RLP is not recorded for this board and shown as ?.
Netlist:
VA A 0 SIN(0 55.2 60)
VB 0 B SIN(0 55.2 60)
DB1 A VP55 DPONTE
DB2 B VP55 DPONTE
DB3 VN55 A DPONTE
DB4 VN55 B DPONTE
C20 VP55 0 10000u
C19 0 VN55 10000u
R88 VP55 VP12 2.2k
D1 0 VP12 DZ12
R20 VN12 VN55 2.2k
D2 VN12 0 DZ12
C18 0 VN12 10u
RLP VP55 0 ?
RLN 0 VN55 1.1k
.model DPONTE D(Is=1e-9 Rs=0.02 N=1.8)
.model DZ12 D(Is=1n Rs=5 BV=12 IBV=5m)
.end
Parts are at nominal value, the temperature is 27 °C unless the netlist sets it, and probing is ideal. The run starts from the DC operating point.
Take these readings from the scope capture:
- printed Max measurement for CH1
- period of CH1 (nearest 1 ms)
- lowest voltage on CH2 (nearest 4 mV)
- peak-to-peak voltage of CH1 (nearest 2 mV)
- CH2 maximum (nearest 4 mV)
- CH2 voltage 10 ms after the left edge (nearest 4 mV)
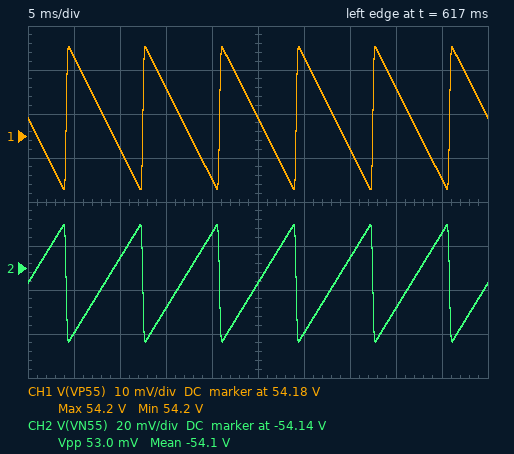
54.2 V
8 ms
-54.172 V
32 mV
-54.120 V
-54.136 V
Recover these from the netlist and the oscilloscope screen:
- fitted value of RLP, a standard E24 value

2.4 kΩ
